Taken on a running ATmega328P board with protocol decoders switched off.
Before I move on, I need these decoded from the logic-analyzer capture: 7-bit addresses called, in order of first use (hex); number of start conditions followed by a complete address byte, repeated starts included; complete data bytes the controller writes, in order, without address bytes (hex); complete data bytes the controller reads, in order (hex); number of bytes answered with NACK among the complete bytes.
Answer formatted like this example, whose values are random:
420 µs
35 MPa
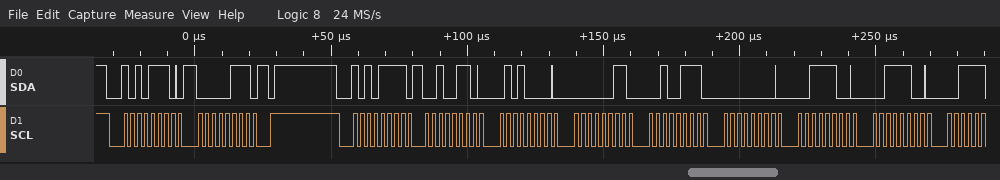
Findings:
0x57
2
07
26 50 03 27 00 3C 3C
0
